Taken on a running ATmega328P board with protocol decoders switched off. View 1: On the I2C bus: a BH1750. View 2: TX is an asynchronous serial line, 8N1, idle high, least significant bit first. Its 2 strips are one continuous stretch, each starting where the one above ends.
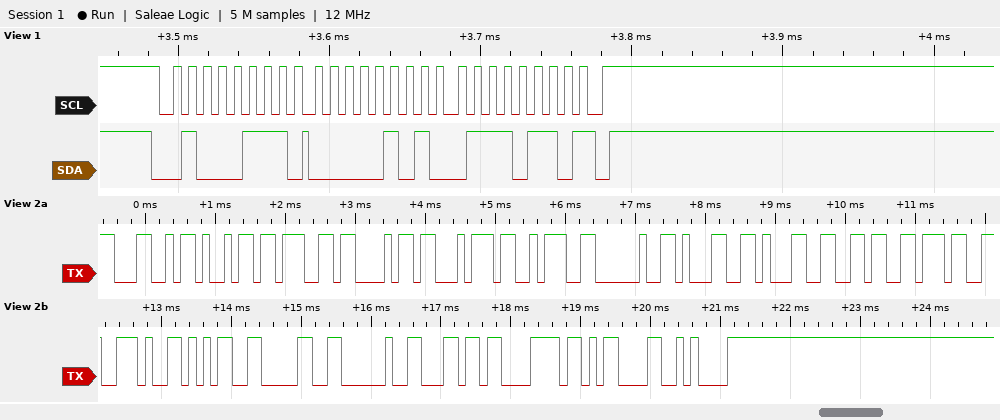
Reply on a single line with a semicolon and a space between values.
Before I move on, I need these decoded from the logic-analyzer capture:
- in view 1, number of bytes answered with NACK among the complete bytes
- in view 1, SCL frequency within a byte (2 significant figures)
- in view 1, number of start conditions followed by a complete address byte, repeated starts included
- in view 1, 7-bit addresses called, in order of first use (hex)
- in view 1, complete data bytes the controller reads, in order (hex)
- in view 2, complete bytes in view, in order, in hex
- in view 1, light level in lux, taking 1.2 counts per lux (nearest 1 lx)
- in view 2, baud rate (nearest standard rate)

1; 100 kHz; 1; 0x23; 05 76; 4C 69 67 68 74 3A 20 31 31 36 37 2E 35 30 20 6C 78 0D 0A; 1165 lx; 9600 baud
